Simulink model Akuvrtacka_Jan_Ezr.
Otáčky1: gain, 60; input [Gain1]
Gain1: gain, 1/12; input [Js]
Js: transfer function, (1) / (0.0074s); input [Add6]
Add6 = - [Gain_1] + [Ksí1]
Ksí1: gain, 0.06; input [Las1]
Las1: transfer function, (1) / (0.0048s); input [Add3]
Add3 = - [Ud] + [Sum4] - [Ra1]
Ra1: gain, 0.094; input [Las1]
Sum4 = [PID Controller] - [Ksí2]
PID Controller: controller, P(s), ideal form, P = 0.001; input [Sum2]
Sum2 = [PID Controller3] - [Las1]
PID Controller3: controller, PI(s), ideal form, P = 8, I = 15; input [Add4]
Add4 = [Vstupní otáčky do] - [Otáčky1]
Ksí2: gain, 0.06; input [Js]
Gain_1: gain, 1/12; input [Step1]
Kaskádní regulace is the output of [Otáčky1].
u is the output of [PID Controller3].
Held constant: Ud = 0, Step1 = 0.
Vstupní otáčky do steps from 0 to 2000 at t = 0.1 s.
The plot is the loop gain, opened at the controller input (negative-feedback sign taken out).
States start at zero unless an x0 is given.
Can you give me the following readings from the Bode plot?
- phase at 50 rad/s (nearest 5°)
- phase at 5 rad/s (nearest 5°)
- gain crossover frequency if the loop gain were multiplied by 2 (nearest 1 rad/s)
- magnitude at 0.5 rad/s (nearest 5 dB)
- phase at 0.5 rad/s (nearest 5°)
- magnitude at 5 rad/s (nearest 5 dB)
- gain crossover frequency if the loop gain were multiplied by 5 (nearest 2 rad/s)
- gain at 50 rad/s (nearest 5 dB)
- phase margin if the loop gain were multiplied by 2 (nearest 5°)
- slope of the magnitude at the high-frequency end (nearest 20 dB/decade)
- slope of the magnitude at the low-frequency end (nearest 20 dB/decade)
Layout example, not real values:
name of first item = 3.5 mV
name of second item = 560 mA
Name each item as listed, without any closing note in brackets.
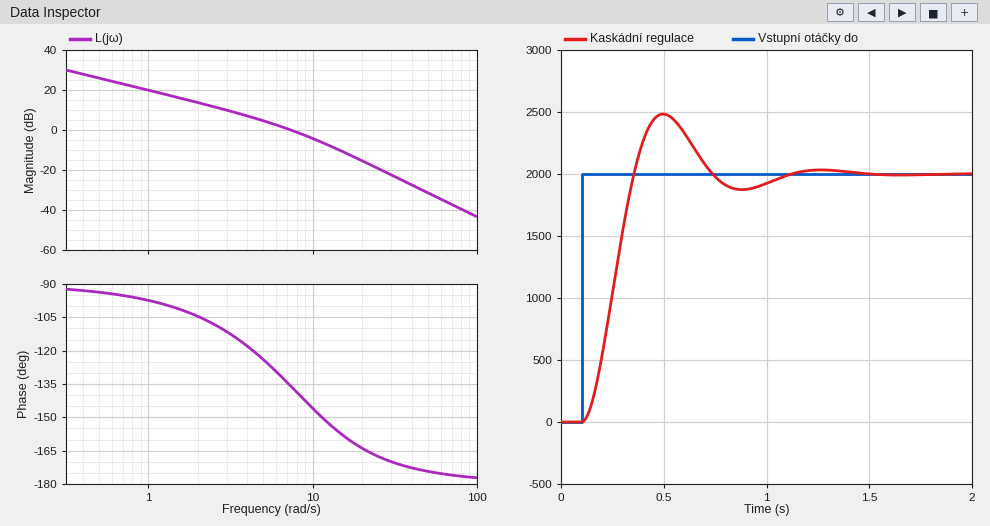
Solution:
phase at 50 rad/s = -175°
phase at 5 rad/s = -125°
gain crossover frequency if the loop gain were multiplied by 2 = 11 rad/s
magnitude at 0.5 rad/s = 25 dB
phase at 0.5 rad/s = -95°
magnitude at 5 rad/s = 5 dB
gain crossover frequency if the loop gain were multiplied by 5 = 18 rad/s
gain at 50 rad/s = -30 dB
phase margin if the loop gain were multiplied by 2 = 30°
slope of the magnitude at the high-frequency end = -40 dB/decade
slope of the magnitude at the low-frequency end = -20 dB/decade
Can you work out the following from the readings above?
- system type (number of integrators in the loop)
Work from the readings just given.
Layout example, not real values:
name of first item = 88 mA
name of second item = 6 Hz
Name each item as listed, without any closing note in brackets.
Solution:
system type = 1
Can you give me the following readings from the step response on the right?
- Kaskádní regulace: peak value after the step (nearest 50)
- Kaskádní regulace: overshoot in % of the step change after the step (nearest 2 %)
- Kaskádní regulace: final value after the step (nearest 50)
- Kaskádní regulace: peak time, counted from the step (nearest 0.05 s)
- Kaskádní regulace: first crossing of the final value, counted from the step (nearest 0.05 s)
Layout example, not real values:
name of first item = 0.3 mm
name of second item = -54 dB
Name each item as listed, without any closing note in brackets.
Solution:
Kaskádní regulace: peak value after the step = 2500
Kaskádní regulace: overshoot in % of the step change after the step = 24 %
Kaskádní regulace: final value after the step = 2000
Kaskádní regulace: peak time, counted from the step = 0.40 s
Kaskádní regulace: first crossing of the final value, counted from the step = 0.25 s
